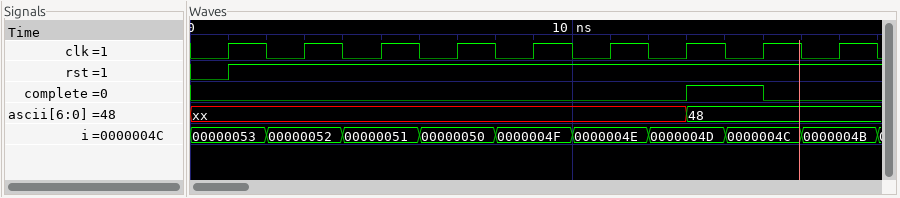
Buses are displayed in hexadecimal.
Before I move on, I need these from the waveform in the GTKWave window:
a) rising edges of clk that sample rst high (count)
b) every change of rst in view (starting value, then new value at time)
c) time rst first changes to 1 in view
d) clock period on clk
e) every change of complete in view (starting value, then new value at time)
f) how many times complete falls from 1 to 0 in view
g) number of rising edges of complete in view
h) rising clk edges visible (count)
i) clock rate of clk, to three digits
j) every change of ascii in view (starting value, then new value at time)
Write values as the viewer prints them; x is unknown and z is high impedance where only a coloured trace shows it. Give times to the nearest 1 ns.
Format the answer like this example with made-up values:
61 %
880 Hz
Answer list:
8
0, 1 at 1 ns
1 ns
2 ns
0, 1 at 13 ns, 0 at 15 ns
1
1
9
500 MHz
xx, 48 at 13 ns
